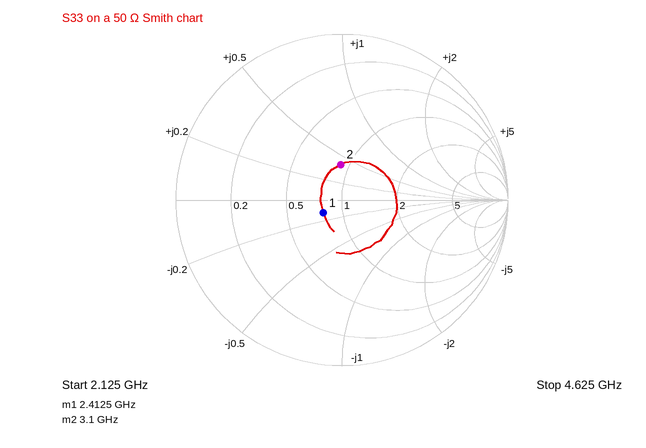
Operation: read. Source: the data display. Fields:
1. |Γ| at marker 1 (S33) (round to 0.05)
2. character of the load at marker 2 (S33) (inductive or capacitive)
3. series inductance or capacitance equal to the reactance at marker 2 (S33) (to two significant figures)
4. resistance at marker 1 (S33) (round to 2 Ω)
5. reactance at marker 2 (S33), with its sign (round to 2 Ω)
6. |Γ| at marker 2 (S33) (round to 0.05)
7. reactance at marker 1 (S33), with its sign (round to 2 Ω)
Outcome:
0.15
inductive
1.0 nH
40 Ω
+20 Ω
0.20
-6 Ω
